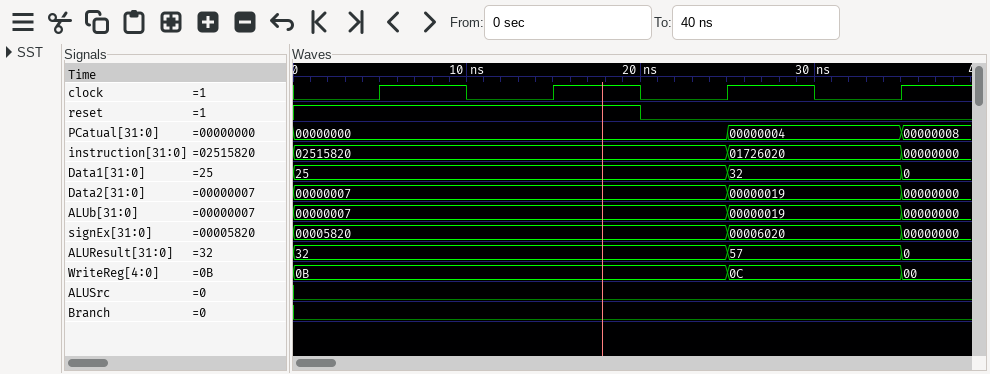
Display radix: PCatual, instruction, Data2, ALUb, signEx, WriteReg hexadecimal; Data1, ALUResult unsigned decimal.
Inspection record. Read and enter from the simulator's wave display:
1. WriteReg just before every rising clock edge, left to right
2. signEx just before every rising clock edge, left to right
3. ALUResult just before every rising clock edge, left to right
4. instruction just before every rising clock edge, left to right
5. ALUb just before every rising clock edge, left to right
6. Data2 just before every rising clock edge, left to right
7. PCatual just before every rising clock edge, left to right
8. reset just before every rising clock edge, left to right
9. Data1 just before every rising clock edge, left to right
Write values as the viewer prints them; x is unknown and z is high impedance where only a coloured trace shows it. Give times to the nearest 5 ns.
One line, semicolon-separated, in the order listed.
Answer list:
0B, 0B, 0B, 0C; 00005820, 00005820, 00005820, 00006020; 32, 32, 32, 57; 02515820, 02515820, 02515820, 01726020; 00000007, 00000007, 00000007, 00000019; 00000007, 00000007, 00000007, 00000019; 00000000, 00000000, 00000000, 00000004; 1 1 0 0; 25, 25, 25, 32
